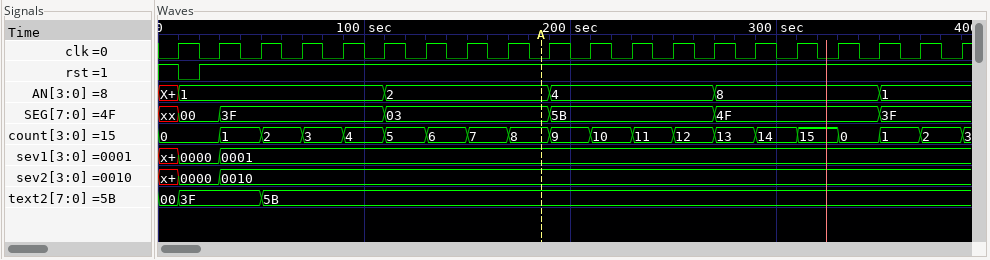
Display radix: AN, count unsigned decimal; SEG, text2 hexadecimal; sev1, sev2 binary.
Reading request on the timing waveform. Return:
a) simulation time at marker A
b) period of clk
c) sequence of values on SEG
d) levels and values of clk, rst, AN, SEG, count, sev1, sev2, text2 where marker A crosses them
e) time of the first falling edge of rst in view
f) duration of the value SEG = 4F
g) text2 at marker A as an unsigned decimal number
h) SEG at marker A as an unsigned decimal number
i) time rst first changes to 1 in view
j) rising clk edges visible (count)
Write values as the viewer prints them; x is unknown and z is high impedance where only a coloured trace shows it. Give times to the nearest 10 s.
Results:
190 s
20 s
xx, 00, 3F, 03, 5B, 4F, 3F
clk=0, rst=1, AN=2, SEG=03, count=8, sev1=0001, sev2=0010, text2=5B
10 s
80 s
91
3
20 s
20
